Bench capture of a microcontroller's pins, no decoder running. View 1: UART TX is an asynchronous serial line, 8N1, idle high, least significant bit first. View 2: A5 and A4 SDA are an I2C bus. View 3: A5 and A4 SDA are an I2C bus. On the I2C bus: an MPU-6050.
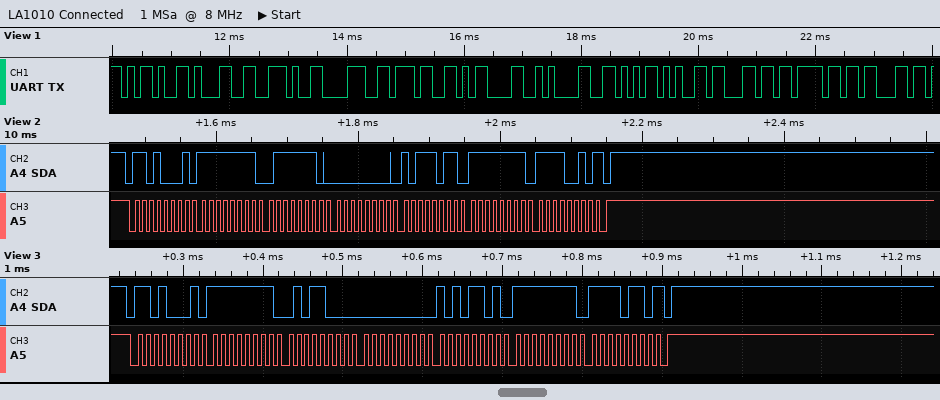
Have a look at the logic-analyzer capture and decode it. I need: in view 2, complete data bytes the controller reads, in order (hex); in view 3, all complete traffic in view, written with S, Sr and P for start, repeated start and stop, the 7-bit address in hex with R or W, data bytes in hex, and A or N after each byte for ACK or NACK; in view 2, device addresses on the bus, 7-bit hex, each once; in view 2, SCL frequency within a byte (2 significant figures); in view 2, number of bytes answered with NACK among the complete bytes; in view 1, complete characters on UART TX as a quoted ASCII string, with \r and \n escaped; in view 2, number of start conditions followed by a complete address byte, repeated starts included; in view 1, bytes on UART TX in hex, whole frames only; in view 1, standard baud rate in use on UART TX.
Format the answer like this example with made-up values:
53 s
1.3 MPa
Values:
FF 7E 00 BB FF F2
S 68R A FF A 58 A 00 A AD A FF A F6 N P
0x68
100 kHz
1
"-1.87\r\nVeloc"
1
0x2D 0x31 0x2E 0x38 0x37 0x0D 0x0A 0x56 0x65 0x6C 0x6F 0x63
9600 baud
